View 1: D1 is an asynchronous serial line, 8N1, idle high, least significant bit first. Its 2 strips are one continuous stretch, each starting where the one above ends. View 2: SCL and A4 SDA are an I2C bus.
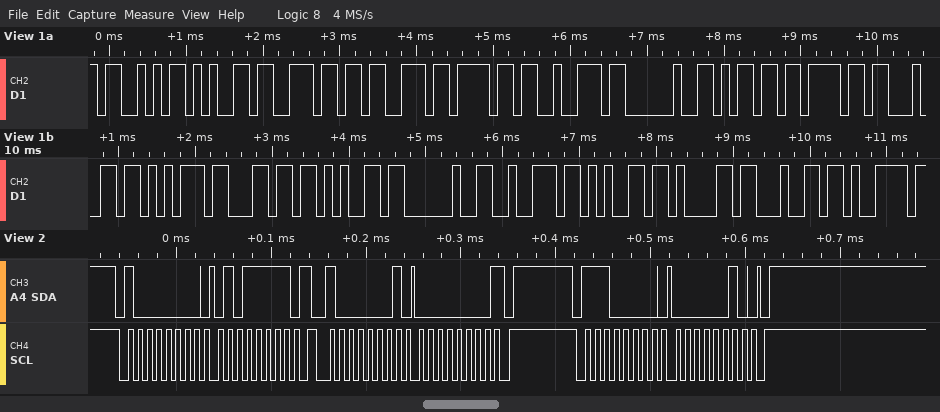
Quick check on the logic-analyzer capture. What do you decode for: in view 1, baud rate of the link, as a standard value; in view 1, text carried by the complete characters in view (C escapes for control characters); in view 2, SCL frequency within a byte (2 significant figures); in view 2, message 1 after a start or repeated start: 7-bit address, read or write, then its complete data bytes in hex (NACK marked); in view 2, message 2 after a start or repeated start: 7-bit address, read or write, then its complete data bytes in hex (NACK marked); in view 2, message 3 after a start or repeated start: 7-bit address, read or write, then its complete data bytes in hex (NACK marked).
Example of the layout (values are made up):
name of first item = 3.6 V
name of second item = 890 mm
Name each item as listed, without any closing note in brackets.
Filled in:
in view 1, baud rate of the link, as a standard value = 9600 baud
in view 1, text carried by the complete characters in view = "Sensor module ready"
in view 2, SCL frequency within a byte = 100 kHz
in view 2, message 1 after a start or repeated start: 7-bit address, read or write, then its complete data bytes in hex = 0x40 write: 5F
in view 2, message 2 after a start or repeated start: 7-bit address, read or write, then its complete data bytes in hex = 0x40 read: 00 NACK
in view 2, message 3 after a start or repeated start: 7-bit address, read or write, then its complete data bytes in hex = 0x70 write: 02
